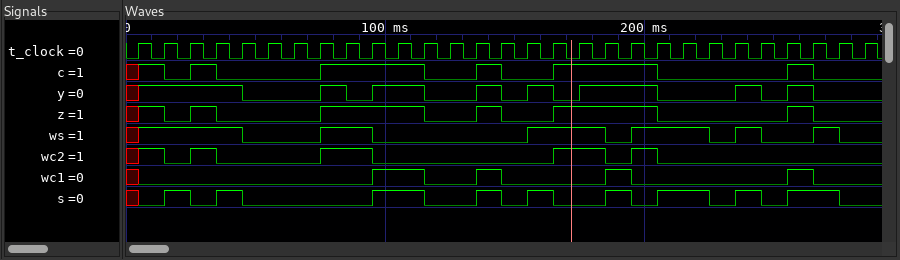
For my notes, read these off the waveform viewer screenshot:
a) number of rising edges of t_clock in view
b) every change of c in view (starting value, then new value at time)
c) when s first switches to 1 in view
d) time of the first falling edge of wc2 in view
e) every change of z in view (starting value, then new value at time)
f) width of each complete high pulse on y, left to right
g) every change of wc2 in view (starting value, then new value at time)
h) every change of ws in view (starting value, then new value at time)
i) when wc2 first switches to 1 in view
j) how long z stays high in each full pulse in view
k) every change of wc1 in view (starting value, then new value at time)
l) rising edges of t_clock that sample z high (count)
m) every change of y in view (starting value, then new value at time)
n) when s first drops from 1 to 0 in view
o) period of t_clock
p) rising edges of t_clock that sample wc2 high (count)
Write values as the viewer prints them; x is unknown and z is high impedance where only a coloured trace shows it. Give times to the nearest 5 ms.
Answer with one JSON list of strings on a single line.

["29", "x, 1 at 5 ms, 0 at 15 ms, 1 at 25 ms, 0 at 35 ms, 1 at 75 ms, 0 at 115 ms, 1 at 135 ms, 0 at 145 ms, 1 at 165 ms, 0 at 205 ms, 1 at 255 ms, 0 at 265 ms", "15 ms", "15 ms", "x, 1 at 5 ms, 0 at 15 ms, 1 at 25 ms, 0 at 35 ms, 1 at 75 ms, 0 at 115 ms, 1 at 135 ms, 0 at 145 ms, 1 at 165 ms, 0 at 205 ms, 1 at 255 ms, 0 at 265 ms", "10 ms, 20 ms, 10 ms, 10 ms, 30 ms, 10 ms, 10 ms", "x, 1 at 5 ms, 0 at 15 ms, 1 at 25 ms, 0 at 35 ms, 1 at 75 ms, 0 at 95 ms, 1 at 165 ms, 0 at 185 ms, 1 at 195 ms, 0 at 205 ms", "x, 1 at 5 ms, 0 at 45 ms, 1 at 75 ms, 0 at 95 ms, 1 at 155 ms, 0 at 185 ms, 1 at 195 ms, 0 at 225 ms, 1 at 235 ms, 0 at 245 ms, 1 at 265 ms, 0 at 275 ms", "5 ms", "10 ms, 40 ms, 10 ms, 40 ms, 10 ms", "x, 0 at 5 ms, 1 at 95 ms, 0 at 115 ms, 1 at 135 ms, 0 at 145 ms, 1 at 185 ms, 0 at 195 ms, 1 at 255 ms, 0 at 265 ms", "12", "x, 1 at 5 ms, 0 at 45 ms, 1 at 75 ms, 0 at 85 ms, 1 at 95 ms, 0 at 115 ms, 1 at 135 ms, 0 at 145 ms, 1 at 155 ms, 0 at 165 ms, 1 at 175 ms, 0 at 205 ms, 1 at 235 ms, 0 at 245 ms, 1 at 255 ms, 0 at 265 ms", "25 ms", "10 ms", "7"]
